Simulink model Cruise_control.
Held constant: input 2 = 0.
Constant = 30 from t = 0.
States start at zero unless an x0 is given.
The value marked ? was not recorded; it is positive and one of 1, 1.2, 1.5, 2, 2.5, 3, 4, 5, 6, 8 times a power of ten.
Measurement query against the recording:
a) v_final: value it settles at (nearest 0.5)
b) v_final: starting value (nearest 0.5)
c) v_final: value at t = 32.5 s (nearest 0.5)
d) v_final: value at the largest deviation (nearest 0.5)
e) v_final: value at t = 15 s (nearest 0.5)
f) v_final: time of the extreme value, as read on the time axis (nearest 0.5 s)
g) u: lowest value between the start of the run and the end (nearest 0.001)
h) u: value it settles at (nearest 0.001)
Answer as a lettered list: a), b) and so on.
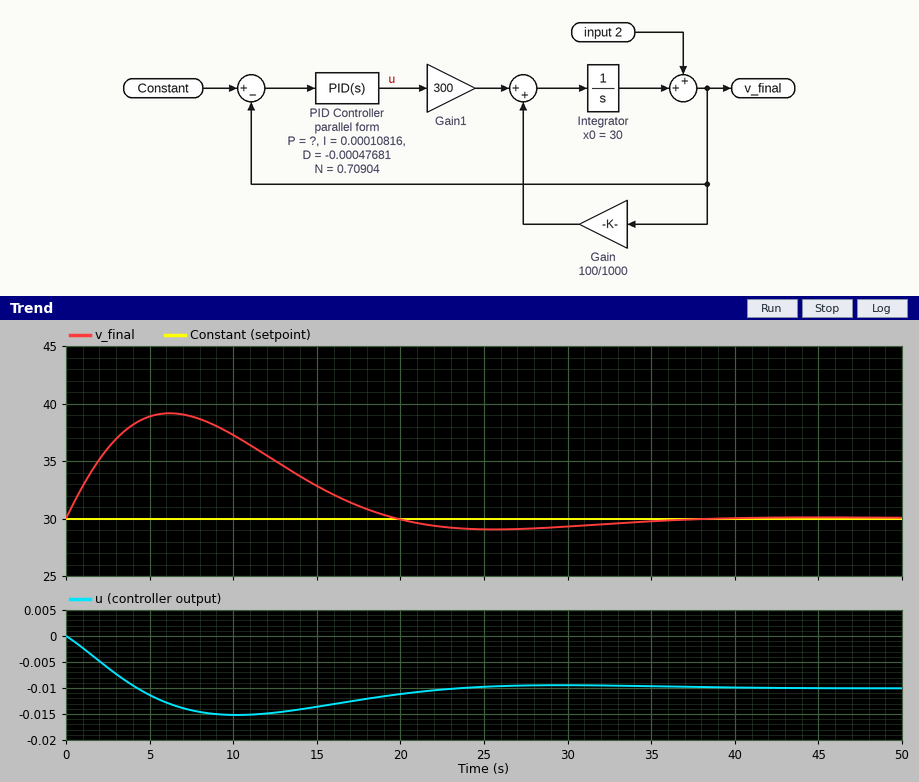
a) 30.0
b) 30.0
c) 29.5
d) 39.0
e) 33.0
f) 6.0 s
g) -0.015
h) -0.010
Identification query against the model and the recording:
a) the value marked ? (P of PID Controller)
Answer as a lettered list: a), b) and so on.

a) 0.001
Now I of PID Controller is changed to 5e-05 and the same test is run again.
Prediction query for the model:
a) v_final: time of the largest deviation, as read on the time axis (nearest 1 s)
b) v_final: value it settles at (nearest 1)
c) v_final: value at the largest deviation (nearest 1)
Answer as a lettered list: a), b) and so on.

a) 8 s
b) 30
c) 41
